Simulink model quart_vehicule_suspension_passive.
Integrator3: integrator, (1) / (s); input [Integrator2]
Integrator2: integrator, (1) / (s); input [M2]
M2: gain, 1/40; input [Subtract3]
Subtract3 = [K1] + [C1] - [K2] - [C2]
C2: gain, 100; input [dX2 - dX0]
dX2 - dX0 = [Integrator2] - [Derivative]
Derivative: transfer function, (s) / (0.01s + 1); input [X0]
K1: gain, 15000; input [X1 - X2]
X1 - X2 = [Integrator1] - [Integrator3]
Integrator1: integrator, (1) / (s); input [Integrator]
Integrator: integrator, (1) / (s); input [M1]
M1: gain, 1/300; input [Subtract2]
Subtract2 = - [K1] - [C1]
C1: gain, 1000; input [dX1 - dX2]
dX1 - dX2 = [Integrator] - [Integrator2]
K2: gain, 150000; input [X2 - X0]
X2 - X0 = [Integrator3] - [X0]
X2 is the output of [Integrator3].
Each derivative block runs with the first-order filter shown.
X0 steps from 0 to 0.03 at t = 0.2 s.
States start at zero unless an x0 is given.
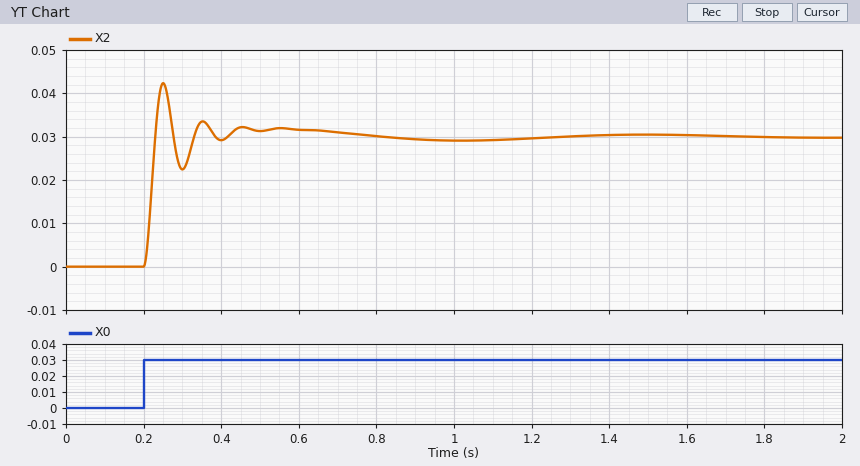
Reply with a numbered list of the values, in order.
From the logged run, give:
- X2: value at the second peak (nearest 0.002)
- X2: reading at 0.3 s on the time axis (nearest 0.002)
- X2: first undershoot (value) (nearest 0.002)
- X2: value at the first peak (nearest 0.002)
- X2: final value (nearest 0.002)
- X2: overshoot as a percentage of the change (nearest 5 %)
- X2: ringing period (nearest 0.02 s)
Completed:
1. 0.034
2. 0.022
3. 0.022
4. 0.042
5. 0.030
6. 40 %
7. 0.10 s
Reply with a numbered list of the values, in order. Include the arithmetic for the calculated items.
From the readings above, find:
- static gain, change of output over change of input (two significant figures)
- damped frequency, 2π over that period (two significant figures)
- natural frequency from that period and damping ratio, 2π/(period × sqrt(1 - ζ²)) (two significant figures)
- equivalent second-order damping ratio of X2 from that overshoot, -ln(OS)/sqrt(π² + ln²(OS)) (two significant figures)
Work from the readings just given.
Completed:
1. (0.03 - 0) / (0.03 - 0) = 1.0
2. 2π / 0.1 = 63 rad/s
3. 2π / (0.1 × sqrt(1 - 0.28²)) = 65 rad/s
4. ln(0.4) = -0.916; 0.916 / sqrt(9.870 + 0.840) = 0.28
